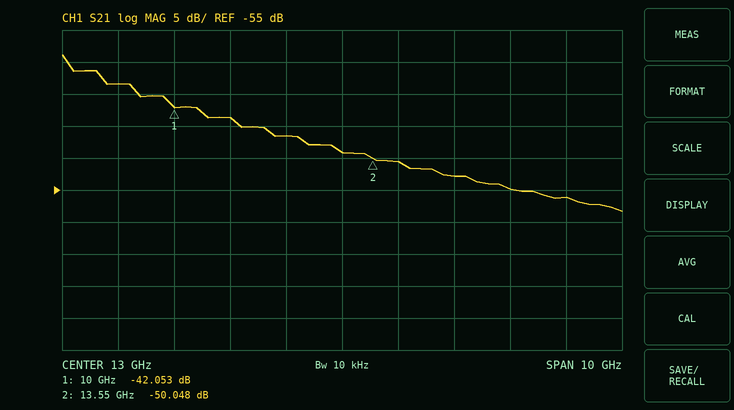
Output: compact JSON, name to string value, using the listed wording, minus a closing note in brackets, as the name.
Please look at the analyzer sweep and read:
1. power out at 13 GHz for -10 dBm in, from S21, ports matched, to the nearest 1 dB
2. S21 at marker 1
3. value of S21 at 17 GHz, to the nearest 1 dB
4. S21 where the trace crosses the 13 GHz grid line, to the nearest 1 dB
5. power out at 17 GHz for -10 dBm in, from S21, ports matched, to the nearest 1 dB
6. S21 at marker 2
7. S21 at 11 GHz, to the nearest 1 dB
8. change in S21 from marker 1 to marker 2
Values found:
{"power out at 13 GHz for -10 dBm in, from S21, ports matched, to the nearest 1 dB": "-59 dBm", "S21 at marker 1": "-42.053 dB", "value of S21 at 17 GHz, to the nearest 1 dB": "-56 dB", "S21 where the trace crosses the 13 GHz grid line, to the nearest 1 dB": "-49 dB", "power out at 17 GHz for -10 dBm in, from S21, ports matched, to the nearest 1 dB": "-66 dBm", "S21 at marker 2": "-50.048 dB", "S21 at 11 GHz, to the nearest 1 dB": "-44 dB", "change in S21 from marker 1 to marker 2": "-7.995 dB"}
